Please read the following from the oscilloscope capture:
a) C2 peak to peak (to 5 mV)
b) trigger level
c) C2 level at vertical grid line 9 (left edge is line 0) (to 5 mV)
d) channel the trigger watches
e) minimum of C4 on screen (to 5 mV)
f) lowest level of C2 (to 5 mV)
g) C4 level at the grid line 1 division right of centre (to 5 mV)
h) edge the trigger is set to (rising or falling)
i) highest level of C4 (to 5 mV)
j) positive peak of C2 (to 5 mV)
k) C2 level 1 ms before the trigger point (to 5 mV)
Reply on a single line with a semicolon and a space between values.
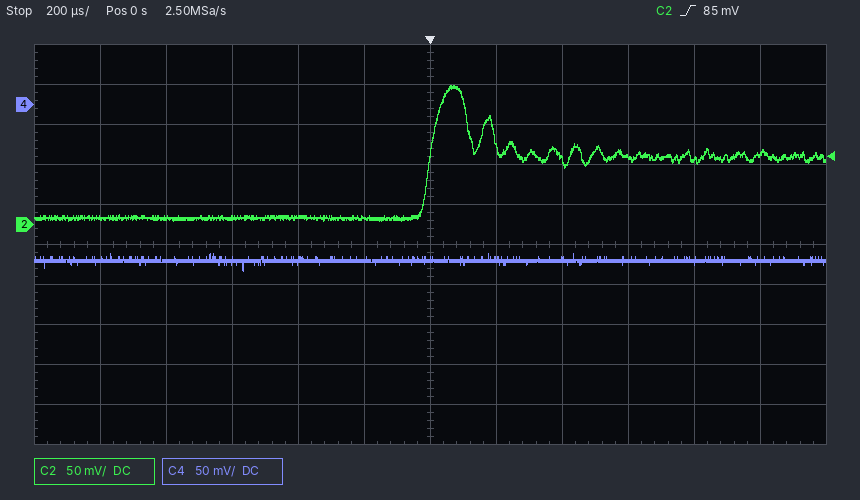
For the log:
170 mV; 85 mV; 85 mV; C2; -210 mV; 5 mV; -195 mV; rising; -185 mV; 175 mV; 10 mV
